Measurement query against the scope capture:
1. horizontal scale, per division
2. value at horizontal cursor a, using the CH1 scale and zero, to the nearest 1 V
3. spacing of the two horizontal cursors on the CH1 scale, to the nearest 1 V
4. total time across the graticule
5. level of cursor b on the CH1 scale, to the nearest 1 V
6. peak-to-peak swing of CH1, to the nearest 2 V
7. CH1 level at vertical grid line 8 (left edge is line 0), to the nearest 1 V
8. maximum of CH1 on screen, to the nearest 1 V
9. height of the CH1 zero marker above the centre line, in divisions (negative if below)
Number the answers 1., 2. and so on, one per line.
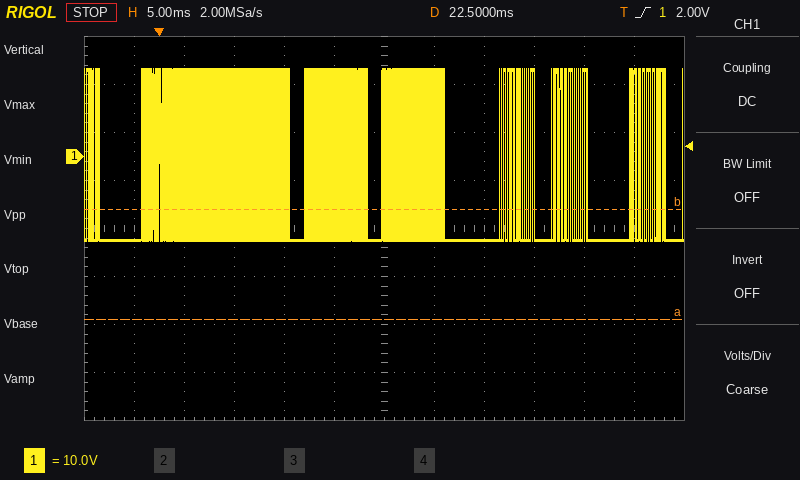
1. 5 ms
2. -34 V
3. 23 V
4. 60 ms
5. -11 V
6. 36 V
7. -17 V
8. 18 V
9. +1.5 div
